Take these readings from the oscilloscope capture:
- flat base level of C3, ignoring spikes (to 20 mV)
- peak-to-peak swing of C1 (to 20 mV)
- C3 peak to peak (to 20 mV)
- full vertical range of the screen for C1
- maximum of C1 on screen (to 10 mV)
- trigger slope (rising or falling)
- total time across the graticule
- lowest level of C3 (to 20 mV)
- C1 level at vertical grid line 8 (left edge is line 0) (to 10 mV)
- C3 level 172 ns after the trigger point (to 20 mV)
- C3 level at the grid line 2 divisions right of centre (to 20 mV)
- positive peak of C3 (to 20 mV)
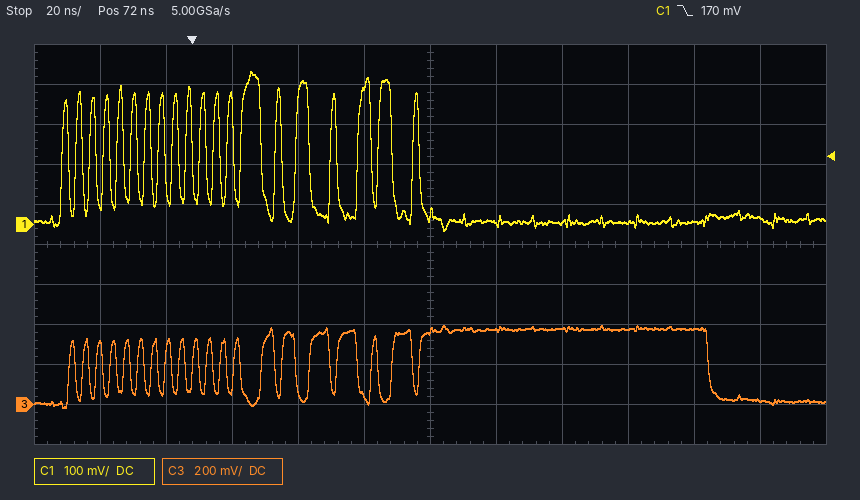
20 mV
400 mV
420 mV
1 V
380 mV
falling
240 ns
-20 mV
10 mV
20 mV
380 mV
400 mV
